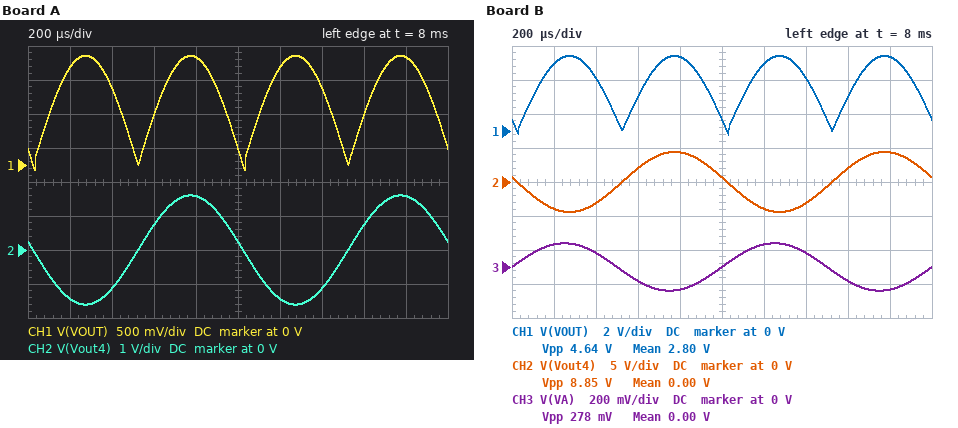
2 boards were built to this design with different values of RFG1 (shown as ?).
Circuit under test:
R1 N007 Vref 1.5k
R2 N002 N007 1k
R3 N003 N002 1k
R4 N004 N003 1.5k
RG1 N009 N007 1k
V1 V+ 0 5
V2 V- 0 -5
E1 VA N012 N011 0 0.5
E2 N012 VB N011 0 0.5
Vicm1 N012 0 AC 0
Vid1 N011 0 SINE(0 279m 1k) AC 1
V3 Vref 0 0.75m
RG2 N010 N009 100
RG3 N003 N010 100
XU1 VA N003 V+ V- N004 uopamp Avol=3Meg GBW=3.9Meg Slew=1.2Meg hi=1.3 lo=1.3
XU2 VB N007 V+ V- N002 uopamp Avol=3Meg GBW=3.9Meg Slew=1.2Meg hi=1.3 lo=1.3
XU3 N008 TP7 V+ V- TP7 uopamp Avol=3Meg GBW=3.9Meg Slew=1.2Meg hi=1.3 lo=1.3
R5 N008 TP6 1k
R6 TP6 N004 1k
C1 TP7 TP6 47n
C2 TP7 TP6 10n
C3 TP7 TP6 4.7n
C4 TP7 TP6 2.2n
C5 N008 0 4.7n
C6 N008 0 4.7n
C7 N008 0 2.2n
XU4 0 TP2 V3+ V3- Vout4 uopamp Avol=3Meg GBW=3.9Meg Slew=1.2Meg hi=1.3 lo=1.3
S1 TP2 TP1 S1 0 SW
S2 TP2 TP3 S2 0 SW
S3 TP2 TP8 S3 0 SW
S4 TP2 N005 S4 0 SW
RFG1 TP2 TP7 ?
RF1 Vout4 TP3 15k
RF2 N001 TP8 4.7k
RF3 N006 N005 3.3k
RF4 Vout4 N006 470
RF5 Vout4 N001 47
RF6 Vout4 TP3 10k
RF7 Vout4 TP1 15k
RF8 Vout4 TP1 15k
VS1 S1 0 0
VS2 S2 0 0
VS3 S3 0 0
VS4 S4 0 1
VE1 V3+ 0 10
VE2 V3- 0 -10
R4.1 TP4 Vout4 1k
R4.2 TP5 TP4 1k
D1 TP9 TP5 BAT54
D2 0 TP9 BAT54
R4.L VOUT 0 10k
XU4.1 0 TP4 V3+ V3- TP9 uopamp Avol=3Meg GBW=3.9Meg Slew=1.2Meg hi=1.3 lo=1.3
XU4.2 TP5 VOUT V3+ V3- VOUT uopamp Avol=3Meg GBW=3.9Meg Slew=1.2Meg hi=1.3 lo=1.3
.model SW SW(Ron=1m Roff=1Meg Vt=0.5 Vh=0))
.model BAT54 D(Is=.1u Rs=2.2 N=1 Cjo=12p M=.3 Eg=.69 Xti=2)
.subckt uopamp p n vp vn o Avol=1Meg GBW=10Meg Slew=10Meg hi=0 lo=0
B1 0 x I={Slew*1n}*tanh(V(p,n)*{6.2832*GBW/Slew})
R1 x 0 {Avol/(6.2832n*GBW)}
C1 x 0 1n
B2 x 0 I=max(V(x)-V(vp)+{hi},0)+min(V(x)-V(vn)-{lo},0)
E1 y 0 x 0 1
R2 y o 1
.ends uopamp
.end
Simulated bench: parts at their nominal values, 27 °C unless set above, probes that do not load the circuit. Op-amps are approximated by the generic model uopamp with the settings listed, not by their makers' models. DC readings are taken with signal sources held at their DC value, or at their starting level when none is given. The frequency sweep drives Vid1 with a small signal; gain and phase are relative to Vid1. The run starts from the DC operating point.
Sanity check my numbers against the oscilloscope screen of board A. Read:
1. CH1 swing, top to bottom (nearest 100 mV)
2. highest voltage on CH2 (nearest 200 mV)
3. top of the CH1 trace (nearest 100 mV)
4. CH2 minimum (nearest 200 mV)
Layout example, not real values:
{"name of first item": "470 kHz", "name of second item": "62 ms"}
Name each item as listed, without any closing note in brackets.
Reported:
{"CH1 swing, top to bottom": "1.7 V", "highest voltage on CH2": "1.6 V", "top of the CH1 trace": "1.6 V", "CH2 minimum": "-1.6 V"}
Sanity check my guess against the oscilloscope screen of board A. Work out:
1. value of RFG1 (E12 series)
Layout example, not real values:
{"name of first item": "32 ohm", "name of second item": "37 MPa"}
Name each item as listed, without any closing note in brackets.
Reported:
{"value of RFG1": "3.3 kΩ"}
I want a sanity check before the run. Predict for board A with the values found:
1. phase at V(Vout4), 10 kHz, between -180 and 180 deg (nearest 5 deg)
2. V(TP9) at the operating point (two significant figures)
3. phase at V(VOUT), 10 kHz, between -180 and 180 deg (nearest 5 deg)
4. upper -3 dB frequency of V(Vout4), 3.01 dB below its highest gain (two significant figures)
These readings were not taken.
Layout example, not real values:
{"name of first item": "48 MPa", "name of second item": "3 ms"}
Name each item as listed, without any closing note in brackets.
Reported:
{"phase at V(Vout4), 10 kHz, between -180 and 180 deg": "25 deg", "V(TP9) at the operating point": "59 mV", "phase at V(VOUT), 10 kHz, between -180 and 180 deg": "-165 deg", "upper -3 dB frequency of V(Vout4), 3.01 dB below its highest gain": "6.9 kHz"}
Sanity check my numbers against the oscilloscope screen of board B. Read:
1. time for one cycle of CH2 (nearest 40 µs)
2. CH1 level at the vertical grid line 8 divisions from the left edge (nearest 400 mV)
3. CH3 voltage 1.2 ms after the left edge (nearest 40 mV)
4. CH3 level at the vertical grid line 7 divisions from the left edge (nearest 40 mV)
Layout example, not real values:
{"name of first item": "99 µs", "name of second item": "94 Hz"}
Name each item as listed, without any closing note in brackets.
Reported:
{"time for one cycle of CH2": "1.00 ms", "CH1 level at the vertical grid line 8 divisions from the left edge": "2.0 V", "CH3 voltage 1.2 ms after the left edge": "120 mV", "CH3 level at the vertical grid line 7 divisions from the left edge": "80 mV"}
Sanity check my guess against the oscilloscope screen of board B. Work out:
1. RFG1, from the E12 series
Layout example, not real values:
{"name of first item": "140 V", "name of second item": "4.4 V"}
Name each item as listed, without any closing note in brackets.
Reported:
{"RFG1, from the E12 series": "1.2 kΩ"}
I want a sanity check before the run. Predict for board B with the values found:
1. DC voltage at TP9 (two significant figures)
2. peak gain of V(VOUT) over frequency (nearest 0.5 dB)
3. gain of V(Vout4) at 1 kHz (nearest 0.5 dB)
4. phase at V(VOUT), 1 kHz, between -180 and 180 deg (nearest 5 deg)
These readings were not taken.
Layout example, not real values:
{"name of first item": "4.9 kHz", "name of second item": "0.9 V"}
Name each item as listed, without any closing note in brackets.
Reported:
{"DC voltage at TP9": "85 mV", "peak gain of V(VOUT) over frequency": "62.5 dB", "gain of V(Vout4) at 1 kHz": "60.5 dB", "phase at V(VOUT), 1 kHz, between -180 and 180 deg": "-10 deg"}
